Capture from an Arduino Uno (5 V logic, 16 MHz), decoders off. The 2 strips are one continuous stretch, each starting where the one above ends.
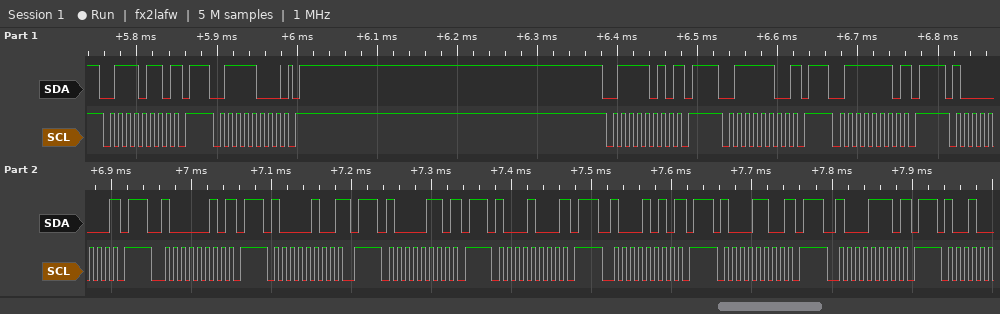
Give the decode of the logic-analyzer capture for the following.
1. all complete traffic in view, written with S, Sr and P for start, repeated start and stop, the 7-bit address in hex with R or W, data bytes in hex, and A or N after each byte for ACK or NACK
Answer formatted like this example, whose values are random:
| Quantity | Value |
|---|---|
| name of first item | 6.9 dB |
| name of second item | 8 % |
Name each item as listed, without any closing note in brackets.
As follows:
| Quantity | Value |
|---|---|
| all complete traffic in view, written with S, Sr and P for start, repeated start and stop, the 7-bit address in hex with R or W, data bytes in hex, and A or N after each byte for ACK or NACK | S 3BW N P S 3CW A P S 3DW N P S 3EW N P S 3FW N P S 40W N P S 41W N P S 42W N P S 43W N P S 44W N P S 45W N P S 46W N P S 47W N P |
